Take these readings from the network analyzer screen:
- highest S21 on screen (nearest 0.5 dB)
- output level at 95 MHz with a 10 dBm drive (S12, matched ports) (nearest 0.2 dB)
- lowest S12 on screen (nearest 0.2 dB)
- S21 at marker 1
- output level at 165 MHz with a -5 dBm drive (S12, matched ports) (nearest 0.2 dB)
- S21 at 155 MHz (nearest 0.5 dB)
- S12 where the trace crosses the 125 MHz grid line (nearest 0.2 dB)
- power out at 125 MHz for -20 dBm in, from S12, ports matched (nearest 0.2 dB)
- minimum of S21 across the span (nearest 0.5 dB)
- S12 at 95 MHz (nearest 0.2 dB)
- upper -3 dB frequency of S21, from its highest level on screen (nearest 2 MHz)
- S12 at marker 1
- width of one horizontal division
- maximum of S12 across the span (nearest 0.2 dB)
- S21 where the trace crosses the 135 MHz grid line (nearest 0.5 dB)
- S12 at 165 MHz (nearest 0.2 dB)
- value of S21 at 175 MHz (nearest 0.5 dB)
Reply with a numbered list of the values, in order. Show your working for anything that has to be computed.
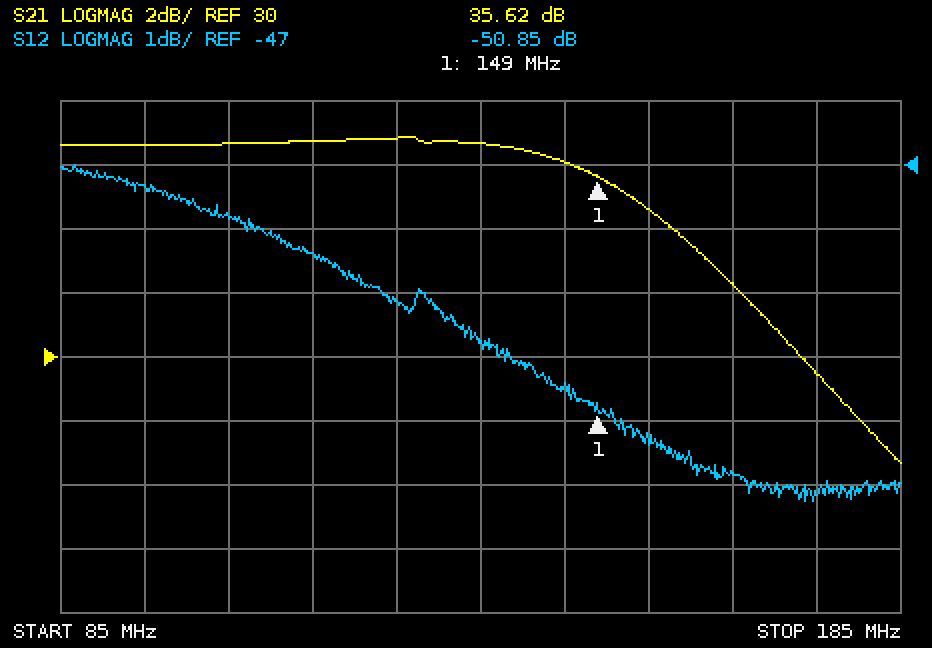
1. 37.0 dB
2. 10 dBm + (-47.4 dB) = -37.4 dBm
3. -52.2 dB
4. 35.62 dB
5. -5 dBm + (-51.8 dB) = -56.8 dBm
6. 34.5 dB
7. -49.2 dB
8. -20 dBm + (-49.2 dB) = -69.2 dBm
9. 26.5 dB
10. -47.4 dB
11. 158 MHz
12. -50.85 dB
13. 10 MHz
14. -47.0 dB
15. 36.5 dB
16. -51.8 dB
17. 29.5 dB
